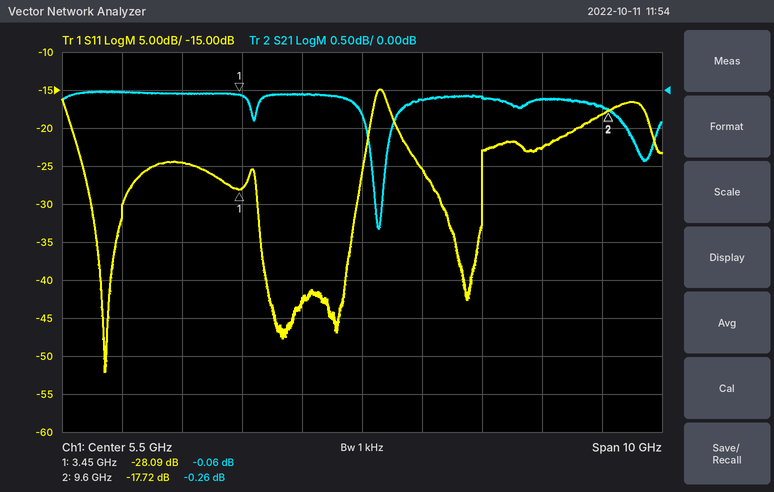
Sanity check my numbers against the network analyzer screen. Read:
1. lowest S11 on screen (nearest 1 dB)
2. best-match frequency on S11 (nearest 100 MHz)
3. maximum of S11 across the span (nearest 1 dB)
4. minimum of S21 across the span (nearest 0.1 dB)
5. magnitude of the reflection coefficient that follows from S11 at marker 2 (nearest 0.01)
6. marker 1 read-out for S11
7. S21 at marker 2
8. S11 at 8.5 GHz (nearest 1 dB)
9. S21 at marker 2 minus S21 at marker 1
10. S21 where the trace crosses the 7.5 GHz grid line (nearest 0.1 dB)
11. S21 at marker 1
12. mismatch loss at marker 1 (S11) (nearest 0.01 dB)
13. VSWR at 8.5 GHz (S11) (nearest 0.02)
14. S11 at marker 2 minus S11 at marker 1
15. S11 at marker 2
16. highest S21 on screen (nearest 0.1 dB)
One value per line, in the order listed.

-52 dB
1.2 GHz
-15 dB
-1.8 dB
0.13
-28.09 dB
-0.26 dB
-23 dB
-0.20 dB
-0.1 dB
-0.06 dB
0.01 dB
1.16
10.37 dB
-17.72 dB
0.0 dB
